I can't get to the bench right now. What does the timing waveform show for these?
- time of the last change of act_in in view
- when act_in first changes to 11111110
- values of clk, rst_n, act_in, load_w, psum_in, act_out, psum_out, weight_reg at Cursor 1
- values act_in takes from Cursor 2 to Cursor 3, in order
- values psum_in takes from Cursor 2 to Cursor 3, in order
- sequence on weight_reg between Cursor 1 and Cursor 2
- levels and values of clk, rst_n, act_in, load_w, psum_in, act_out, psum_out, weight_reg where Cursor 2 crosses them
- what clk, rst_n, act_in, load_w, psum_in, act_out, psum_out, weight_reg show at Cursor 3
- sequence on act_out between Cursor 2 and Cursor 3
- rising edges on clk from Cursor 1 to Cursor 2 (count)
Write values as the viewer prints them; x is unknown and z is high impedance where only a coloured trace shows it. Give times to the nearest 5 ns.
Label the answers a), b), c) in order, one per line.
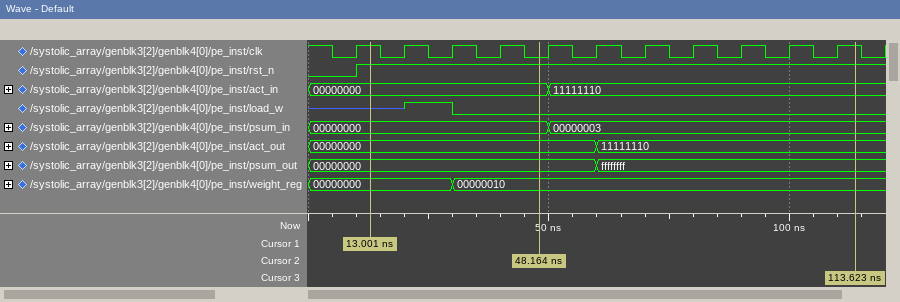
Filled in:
a) 50 ns
b) 50 ns
c) clk=1, rst_n=1, act_in=00000000, load_w=z, psum_in=00000000, act_out=00000000, psum_out=00000000, weight_reg=00000000
d) 00000000, 11111110
e) 00000000, 00000003
f) 00000000, 00000010
g) clk=0, rst_n=1, act_in=00000000, load_w=0, psum_in=00000000, act_out=00000000, psum_out=00000000, weight_reg=00000010
h) clk=1, rst_n=1, act_in=11111110, load_w=0, psum_in=00000003, act_out=11111110, psum_out=ffffffff, weight_reg=00000010
i) 00000000, 11111110
j) 3
